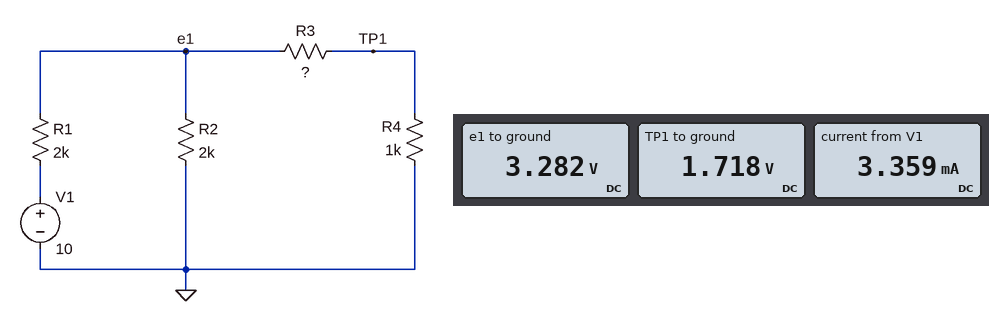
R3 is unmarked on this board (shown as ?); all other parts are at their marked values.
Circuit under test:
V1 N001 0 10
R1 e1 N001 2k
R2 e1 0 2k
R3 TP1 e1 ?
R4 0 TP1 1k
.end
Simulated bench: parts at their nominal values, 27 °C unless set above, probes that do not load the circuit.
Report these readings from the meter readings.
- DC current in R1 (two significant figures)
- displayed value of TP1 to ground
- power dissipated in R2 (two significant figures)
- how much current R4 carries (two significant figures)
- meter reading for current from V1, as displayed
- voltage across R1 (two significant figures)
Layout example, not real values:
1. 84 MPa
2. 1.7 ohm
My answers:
1. 3.4 mA
2. 1.718 V
3. 5.4 mW
4. 1.7 mA
5. 3.359 mA
6. 6.7 V
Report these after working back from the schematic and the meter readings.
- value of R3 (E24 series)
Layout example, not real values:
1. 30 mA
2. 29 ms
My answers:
1. 910 Ω
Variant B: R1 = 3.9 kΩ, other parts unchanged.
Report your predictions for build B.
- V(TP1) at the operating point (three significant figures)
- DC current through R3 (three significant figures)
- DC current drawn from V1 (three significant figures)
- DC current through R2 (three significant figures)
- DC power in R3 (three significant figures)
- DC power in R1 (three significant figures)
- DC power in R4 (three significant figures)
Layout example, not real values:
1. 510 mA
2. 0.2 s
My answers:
1. 1.05 V
2. 1.05 mA
3. 2.05 mA
4. 1.00 mA
5. 1.00 mW
6. 16.4 mW
7. 1.10 mW
